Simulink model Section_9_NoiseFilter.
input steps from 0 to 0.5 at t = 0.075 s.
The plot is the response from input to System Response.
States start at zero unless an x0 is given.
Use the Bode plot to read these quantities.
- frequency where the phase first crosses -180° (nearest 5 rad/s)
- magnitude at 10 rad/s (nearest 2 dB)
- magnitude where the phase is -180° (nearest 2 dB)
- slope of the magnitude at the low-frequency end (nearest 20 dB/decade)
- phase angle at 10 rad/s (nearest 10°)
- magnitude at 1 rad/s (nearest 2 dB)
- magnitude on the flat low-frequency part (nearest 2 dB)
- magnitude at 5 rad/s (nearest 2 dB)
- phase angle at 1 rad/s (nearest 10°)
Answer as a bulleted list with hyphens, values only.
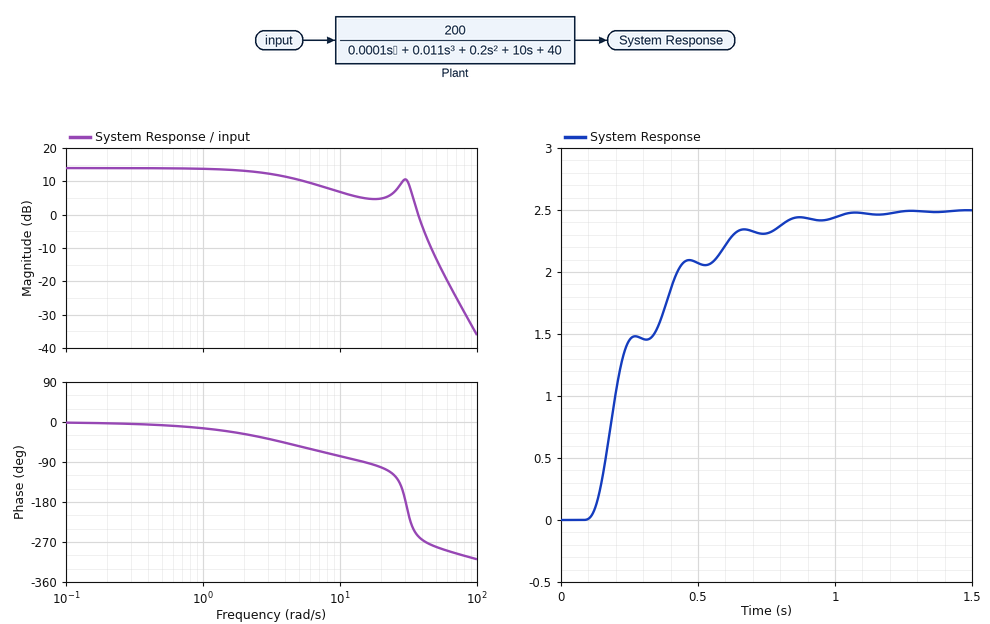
- 30 rad/s
- 6 dB
- 10 dB
- 0 dB/decade
- -80°
- 14 dB
- 14 dB
- 10 dB
- -10°
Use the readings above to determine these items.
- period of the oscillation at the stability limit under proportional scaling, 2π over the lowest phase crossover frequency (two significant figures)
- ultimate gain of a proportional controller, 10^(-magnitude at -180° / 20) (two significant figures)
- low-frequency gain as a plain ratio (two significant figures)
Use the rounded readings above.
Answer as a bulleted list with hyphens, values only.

- 0.21 s
- 0.32
- 5.0
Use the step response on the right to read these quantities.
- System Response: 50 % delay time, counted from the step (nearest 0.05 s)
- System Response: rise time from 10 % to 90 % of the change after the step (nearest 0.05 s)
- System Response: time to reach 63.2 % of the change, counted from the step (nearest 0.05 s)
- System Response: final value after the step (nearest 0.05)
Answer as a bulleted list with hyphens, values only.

- 0.15 s
- 0.45 s
- 0.30 s
- 2.50
